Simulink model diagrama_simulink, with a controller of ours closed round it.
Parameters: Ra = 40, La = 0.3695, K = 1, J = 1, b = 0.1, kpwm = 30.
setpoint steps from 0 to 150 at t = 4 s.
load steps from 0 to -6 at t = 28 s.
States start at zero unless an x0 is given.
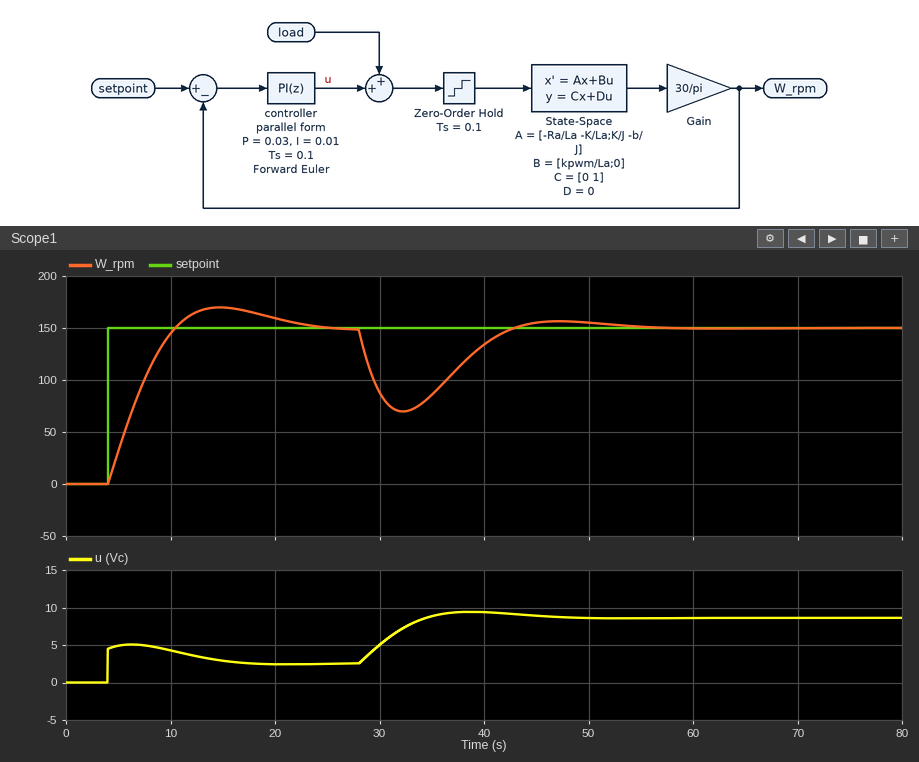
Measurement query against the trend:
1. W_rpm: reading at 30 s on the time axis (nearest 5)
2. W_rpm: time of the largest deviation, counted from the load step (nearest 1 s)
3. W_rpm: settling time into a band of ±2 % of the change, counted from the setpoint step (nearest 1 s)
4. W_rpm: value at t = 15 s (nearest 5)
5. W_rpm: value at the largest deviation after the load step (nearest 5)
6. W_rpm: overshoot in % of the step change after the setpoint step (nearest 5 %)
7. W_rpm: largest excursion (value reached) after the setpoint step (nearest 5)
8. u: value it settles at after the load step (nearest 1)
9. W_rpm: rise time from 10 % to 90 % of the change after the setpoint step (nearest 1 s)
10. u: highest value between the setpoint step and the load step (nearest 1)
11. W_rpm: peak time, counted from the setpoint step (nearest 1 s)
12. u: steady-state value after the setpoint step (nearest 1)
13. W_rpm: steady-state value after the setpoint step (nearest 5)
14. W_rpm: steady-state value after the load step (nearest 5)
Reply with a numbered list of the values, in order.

1. 90
2. 4 s
3. 19 s
4. 170
5. 70
6. 15 %
7. 170
8. 9
9. 5 s
10. 5
11. 11 s
12. 3
13. 150
14. 150
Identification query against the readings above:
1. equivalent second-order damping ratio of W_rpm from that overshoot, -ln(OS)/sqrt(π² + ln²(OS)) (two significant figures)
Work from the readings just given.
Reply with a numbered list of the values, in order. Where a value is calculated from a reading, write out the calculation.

1. ln(0.15) = -1.897; 1.897 / sqrt(9.870 + 3.599) = 0.52
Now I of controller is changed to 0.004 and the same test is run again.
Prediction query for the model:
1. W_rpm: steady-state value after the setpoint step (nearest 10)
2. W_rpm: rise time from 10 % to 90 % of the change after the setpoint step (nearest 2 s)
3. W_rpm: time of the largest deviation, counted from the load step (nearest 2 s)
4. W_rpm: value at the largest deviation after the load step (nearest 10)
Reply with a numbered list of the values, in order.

1. 150
2. 10 s
3. 6 s
4. 60
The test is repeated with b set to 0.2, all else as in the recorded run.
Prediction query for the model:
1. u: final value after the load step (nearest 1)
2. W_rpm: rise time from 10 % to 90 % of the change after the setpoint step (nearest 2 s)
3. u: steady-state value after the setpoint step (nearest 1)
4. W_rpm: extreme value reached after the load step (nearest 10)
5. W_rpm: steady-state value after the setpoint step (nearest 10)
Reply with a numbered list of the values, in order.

1. 11
2. 6 s
3. 5
4. 80
5. 150
